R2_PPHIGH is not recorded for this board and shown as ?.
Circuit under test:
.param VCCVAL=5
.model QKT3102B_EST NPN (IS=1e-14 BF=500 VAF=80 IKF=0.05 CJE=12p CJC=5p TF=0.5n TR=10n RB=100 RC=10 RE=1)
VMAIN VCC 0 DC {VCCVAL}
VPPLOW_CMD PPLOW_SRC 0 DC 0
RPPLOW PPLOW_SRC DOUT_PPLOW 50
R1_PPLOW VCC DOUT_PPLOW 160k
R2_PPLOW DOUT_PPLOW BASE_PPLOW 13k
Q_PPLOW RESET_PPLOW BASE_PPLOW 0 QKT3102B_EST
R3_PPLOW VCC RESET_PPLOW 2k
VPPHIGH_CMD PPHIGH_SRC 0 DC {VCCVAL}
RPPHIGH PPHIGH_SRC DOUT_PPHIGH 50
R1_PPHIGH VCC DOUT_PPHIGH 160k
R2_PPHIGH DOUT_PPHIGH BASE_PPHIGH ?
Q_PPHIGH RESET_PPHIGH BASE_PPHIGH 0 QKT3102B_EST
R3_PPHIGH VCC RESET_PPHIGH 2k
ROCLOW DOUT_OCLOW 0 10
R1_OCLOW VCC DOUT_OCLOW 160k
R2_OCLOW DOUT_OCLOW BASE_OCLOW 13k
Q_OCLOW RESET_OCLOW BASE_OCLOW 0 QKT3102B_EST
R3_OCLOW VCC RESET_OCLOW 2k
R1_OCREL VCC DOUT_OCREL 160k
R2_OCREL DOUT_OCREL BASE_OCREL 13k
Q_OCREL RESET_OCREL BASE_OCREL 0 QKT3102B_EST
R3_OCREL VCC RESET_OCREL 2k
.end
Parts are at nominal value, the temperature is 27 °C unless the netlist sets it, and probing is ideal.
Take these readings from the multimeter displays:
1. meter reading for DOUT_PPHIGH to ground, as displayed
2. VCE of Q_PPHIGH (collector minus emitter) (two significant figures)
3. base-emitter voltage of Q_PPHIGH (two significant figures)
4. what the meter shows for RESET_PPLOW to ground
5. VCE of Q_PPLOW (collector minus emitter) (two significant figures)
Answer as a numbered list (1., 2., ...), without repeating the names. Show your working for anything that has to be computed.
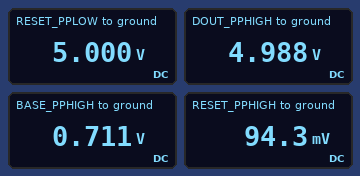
1. 4.988 V
2. 94.3 mV = 94 mV
3. 711 mV = 710 mV
4. 5.000 V
5. 5 V = 5.0 V
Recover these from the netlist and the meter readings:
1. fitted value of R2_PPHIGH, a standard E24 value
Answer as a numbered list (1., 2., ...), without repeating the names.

1. 18 kΩ
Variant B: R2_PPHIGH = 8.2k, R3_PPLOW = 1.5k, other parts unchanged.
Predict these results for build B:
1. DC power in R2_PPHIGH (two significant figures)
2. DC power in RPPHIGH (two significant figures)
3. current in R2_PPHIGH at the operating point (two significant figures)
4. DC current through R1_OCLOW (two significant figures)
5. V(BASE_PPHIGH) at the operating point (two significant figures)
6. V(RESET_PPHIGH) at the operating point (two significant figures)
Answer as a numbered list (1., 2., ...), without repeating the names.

1. 2.2 mW
2. 13 µW
3. 520 µA
4. 31 µA
5. 740 mV
6. 79 mV
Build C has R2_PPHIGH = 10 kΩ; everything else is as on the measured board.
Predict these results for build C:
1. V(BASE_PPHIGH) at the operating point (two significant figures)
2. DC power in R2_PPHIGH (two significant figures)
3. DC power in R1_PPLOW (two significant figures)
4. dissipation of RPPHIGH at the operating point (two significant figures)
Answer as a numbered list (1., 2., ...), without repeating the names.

1. 730 mV
2. 1.8 mW
3. 160 µW
4. 9.0 µW
